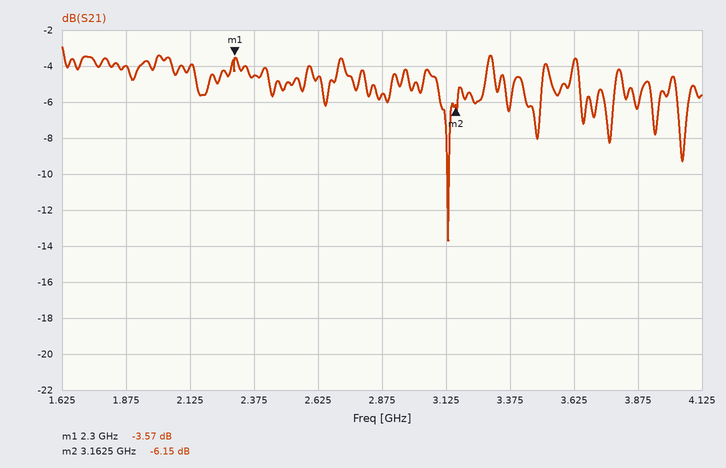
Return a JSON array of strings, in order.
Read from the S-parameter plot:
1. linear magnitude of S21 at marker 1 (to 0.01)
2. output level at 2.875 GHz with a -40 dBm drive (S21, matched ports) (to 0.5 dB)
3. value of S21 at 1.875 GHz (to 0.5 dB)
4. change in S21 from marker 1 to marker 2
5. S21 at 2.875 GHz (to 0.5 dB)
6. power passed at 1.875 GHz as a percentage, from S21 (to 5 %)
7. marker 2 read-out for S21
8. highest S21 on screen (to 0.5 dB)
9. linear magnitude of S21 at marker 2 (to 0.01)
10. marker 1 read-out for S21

["0.66", "-45.5 dBm", "-4.0 dB", "-2.58 dB", "-5.5 dB", "40 %", "-6.15 dB", "-3.0 dB", "0.49", "-3.57 dB"]
